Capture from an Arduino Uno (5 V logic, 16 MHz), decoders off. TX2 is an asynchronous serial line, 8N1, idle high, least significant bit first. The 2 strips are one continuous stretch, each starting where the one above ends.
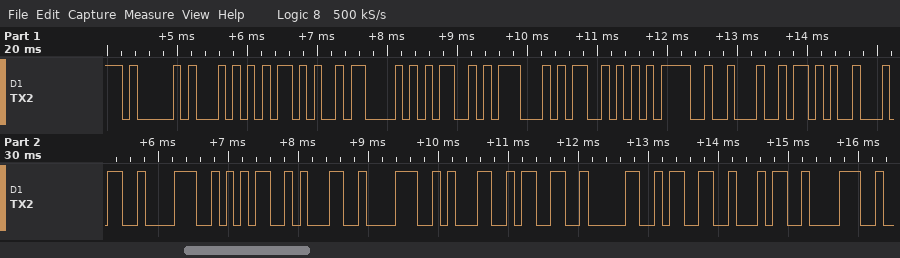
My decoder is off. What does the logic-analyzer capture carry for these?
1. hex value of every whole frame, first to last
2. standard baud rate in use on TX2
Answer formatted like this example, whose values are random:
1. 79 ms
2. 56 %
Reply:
1. 0x41 0x54 0x2B 0x43 0x4D 0x47 0x53 0x3D 0x22 0x2B 0x34 0x38 0x35 0x31 0x38 0x31 0x33 0x30 0x33 0x34 0x38
2. 9600 baud
